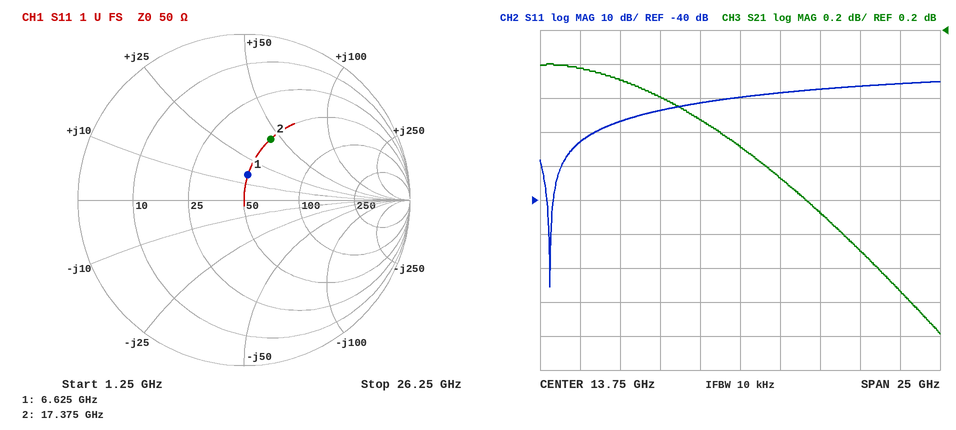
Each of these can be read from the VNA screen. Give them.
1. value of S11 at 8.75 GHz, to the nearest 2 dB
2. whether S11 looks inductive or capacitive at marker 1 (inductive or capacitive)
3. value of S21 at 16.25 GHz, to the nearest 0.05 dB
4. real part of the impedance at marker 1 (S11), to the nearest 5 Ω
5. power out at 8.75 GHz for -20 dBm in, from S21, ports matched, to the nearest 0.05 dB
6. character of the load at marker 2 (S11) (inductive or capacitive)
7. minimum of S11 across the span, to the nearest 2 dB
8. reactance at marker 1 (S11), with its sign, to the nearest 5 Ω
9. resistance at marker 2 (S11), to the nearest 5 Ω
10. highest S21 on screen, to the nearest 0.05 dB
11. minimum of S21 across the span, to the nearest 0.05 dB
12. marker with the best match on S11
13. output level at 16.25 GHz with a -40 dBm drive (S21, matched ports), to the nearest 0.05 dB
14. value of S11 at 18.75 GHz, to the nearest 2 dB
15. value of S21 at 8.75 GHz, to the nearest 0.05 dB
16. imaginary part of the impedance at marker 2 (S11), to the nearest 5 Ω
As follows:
-14 dB
inductive
-0.65 dB
50 Ω
-20.20 dBm
inductive
-66 dB
+15 Ω
50 Ω
0.00 dB
-1.60 dB
marker 1
-40.65 dBm
-8 dB
-0.20 dB
+45 Ω
